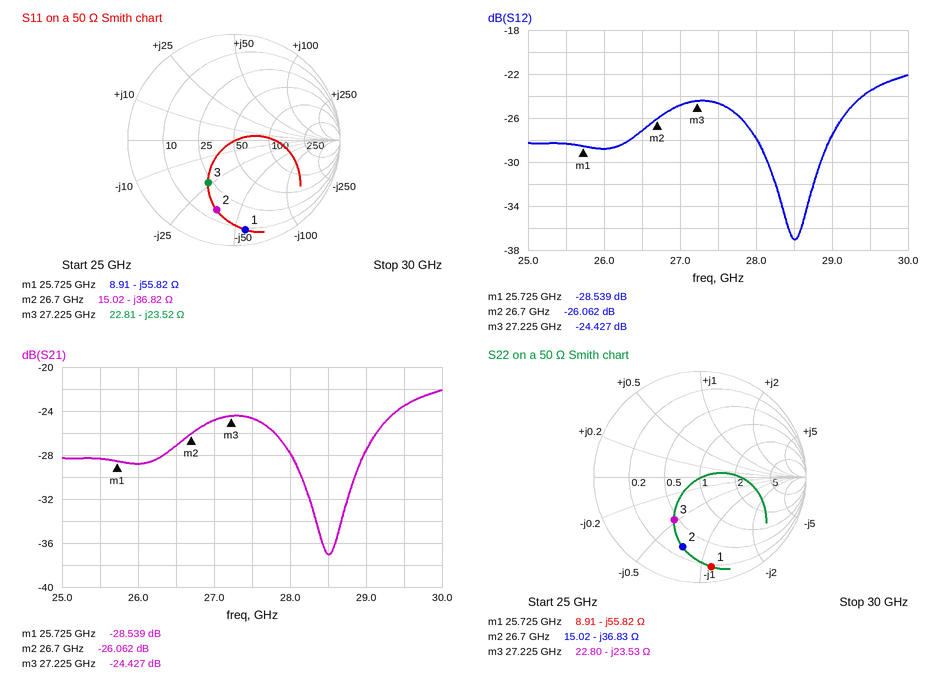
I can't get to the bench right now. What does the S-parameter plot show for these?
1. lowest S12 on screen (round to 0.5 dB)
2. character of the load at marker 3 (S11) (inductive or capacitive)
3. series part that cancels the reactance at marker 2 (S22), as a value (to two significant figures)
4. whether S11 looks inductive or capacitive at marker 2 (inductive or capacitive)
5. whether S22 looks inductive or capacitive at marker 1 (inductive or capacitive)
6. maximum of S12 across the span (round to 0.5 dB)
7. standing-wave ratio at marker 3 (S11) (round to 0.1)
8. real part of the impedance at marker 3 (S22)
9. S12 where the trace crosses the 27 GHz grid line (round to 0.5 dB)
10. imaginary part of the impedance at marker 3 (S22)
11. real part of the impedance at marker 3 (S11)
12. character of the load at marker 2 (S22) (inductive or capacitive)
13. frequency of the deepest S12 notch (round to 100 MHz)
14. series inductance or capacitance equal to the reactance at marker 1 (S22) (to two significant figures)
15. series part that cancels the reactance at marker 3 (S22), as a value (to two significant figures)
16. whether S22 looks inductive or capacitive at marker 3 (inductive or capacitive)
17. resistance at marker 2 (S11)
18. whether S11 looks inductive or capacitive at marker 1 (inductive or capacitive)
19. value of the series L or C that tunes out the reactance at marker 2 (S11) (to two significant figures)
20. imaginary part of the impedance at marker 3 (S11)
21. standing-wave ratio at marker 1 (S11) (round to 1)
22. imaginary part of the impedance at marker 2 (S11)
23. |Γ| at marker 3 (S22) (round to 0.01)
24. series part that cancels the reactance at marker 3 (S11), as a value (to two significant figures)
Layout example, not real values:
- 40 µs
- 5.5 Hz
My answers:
- -37.0 dB
- capacitive
- 220 pH
- capacitive
- capacitive
- -22.0 dB
- 2.8
- 22.80 Ω
- -25.0 dB
- -23.53 Ω
- 22.81 Ω
- capacitive
- 28.5 GHz
- 110 fF
- 140 pH
- capacitive
- 15.02 Ω
- capacitive
- 220 pH
- -23.52 Ω
- 13
- -36.82 Ω
- 0.47
- 140 pH
